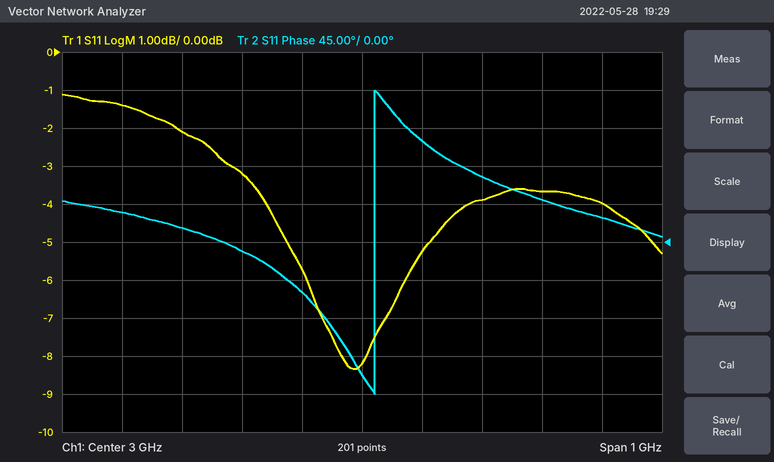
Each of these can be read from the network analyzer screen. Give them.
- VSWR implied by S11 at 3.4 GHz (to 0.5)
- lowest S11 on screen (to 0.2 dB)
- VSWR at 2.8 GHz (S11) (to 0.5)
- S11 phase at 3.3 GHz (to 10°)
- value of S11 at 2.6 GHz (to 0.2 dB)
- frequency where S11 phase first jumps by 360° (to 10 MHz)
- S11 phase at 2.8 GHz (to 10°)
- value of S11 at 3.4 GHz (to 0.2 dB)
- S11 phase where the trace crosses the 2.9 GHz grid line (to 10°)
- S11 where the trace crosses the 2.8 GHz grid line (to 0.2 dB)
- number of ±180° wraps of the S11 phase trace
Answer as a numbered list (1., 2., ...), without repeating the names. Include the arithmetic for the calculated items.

1. |Γ| = 10^(-4/20) = 0.6310; VSWR = (1 + 0.6310)/(1 − 0.6310) ≈ 4.42, so 4.5 to the nearest 0.5
2. -8.4 dB
3. |Γ| = 10^(-3.2/20) = 0.6918; VSWR = (1 + 0.6918)/(1 − 0.6918) ≈ 5.5
4. 50°
5. -1.4 dB
6. 3.02 GHz
7. -10°
8. -4.0 dB
9. -60°
10. -3.2 dB
11. 1
